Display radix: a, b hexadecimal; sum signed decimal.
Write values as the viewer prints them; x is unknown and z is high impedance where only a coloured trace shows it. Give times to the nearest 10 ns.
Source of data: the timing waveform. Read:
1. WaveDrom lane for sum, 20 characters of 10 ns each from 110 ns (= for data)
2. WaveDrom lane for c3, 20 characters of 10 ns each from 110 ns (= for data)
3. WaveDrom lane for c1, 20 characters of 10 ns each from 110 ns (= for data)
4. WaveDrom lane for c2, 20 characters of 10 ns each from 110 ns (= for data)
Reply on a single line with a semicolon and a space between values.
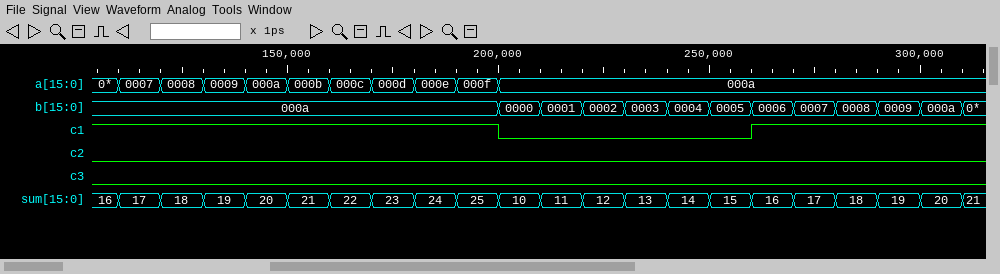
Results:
{name: 'sum', wave: '====================', data: '17 18 19 20 21 22 23 24 25 10 11 12 13 14 15 16 17 18 19 20'}; {name: 'c3', wave: '0...................'}; {name: 'c1', wave: '1........0.....1....'}; {name: 'c2', wave: '0...................'}
